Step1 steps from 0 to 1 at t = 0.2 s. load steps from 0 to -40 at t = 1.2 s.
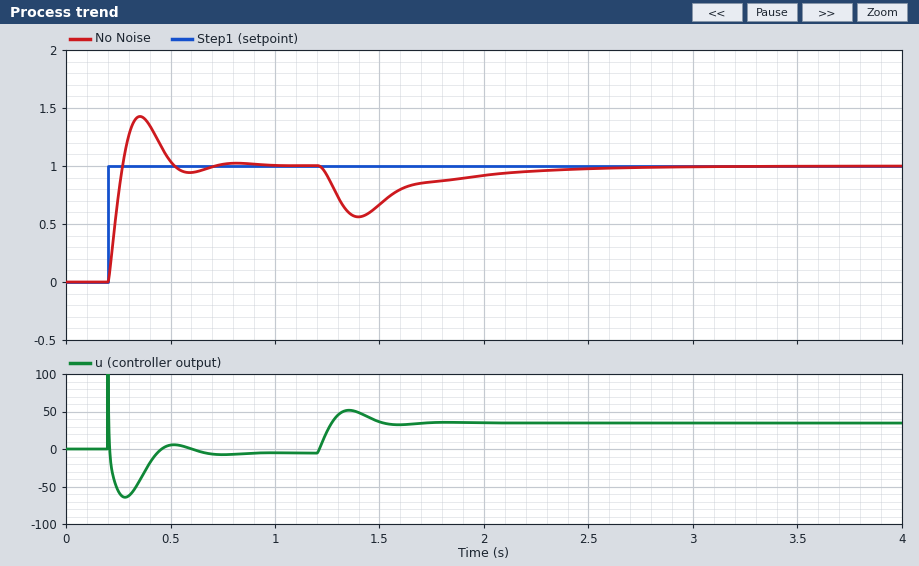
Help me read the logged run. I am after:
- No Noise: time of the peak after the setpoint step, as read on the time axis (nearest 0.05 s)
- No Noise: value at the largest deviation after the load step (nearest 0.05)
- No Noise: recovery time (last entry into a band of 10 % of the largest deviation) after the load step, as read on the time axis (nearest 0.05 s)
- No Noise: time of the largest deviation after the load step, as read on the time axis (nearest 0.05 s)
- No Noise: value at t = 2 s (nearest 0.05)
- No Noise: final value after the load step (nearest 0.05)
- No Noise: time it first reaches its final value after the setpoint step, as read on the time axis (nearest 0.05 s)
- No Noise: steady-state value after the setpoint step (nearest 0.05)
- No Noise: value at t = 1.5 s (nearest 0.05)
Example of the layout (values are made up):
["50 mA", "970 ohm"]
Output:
["0.35 s", "0.55", "2.25 s", "1.40 s", "0.90", "1.00", "0.25 s", "1.00", "0.65"]
